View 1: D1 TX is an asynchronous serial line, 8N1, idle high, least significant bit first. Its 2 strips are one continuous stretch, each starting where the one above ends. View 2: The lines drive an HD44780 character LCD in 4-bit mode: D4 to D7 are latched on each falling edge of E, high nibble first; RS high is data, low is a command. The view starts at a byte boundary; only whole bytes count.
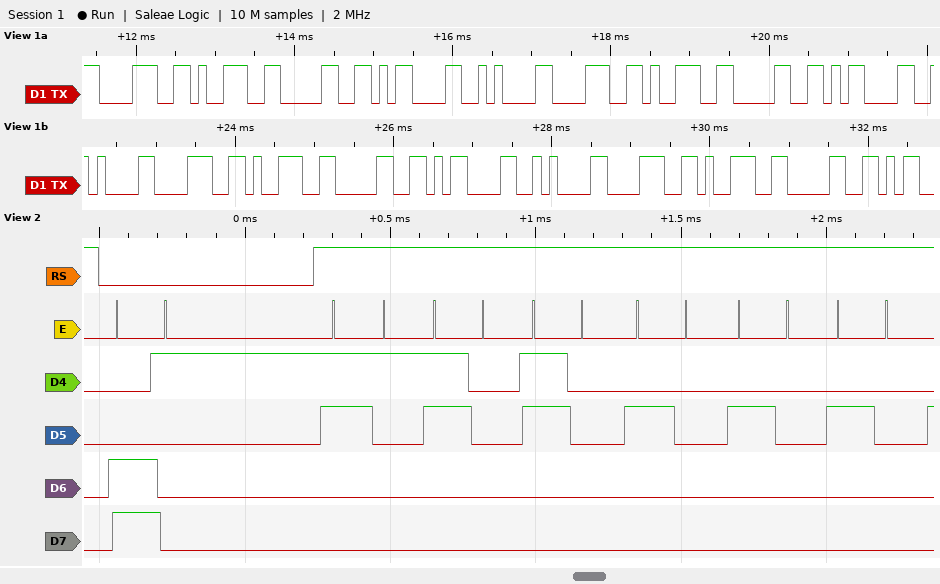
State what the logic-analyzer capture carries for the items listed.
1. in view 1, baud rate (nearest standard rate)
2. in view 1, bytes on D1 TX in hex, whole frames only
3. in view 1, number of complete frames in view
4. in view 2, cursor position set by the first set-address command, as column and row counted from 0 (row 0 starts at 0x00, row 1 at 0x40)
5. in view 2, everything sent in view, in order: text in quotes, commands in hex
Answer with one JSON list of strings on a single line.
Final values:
["9600 baud", "38 39 30 0D 0A 38 39 30 0D 0A 38 39 30 0D 0A 38 39 30", "18", "column 1, row 1", "0xC1 \"100   \""]
